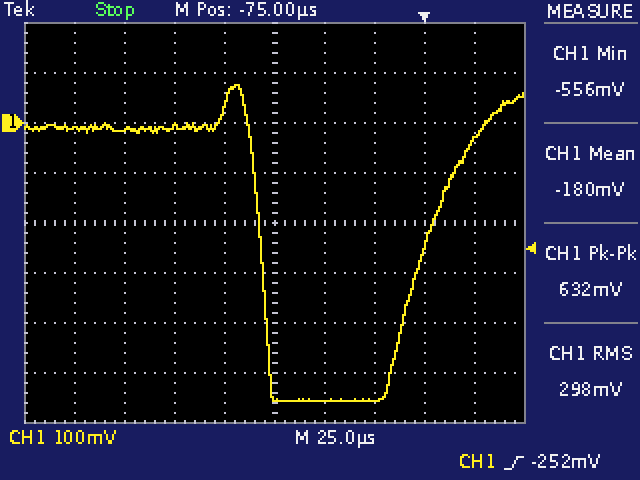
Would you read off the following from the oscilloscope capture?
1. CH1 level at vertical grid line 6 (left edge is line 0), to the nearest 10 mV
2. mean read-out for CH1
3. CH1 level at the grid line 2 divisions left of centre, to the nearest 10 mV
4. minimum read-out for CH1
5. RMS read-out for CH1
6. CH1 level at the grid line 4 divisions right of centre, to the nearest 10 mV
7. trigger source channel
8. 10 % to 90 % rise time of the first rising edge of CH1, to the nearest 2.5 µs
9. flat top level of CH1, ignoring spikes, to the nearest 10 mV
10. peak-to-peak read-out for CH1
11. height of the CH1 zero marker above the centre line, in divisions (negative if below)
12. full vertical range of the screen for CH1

-560 mV
-180 mV
-10 mV
-556 mV
298 mV
-30 mV
CH1
37.5 µs
-10 mV
632 mV
+2.0 div
800 mV
